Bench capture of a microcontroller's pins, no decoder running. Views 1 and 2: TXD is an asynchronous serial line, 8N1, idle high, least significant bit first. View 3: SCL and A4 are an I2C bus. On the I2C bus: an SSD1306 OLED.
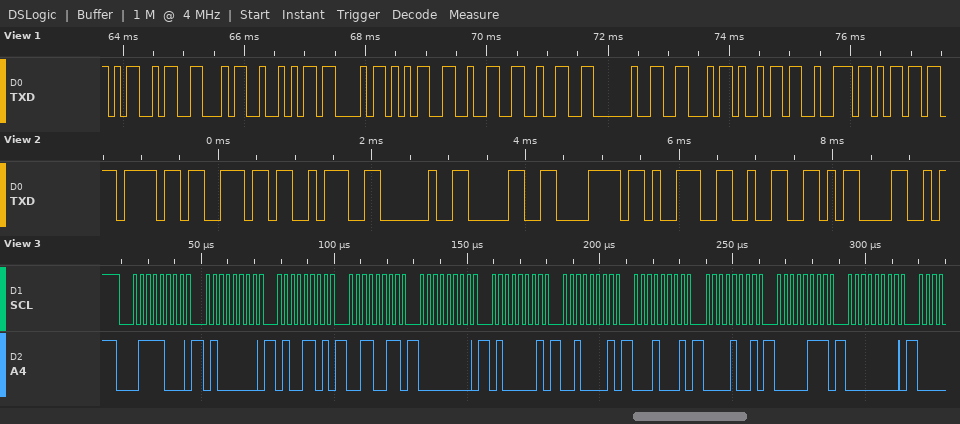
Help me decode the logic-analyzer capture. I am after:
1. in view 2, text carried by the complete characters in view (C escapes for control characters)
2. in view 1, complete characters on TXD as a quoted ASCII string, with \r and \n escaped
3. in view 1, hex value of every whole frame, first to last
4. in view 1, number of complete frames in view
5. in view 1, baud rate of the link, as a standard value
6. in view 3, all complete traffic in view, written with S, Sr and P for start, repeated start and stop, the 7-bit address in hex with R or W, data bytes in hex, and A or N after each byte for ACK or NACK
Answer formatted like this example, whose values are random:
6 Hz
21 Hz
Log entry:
"on: 0x92\r"
"MFRC522 Firm"
4D 46 52 43 35 32 32 20 46 69 72 6D
12
9600 baud
S 3CW A 40 A 4D A 33 A 00 A 41 A 21 A 11 A 09 A 07 A 00 A
